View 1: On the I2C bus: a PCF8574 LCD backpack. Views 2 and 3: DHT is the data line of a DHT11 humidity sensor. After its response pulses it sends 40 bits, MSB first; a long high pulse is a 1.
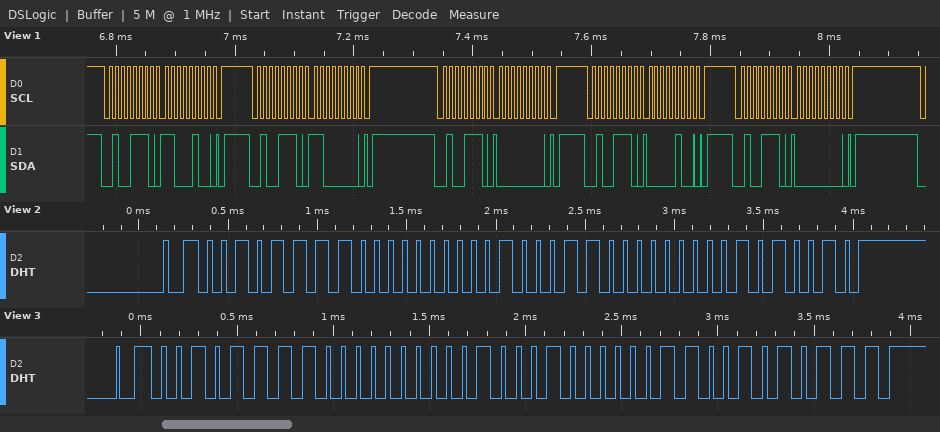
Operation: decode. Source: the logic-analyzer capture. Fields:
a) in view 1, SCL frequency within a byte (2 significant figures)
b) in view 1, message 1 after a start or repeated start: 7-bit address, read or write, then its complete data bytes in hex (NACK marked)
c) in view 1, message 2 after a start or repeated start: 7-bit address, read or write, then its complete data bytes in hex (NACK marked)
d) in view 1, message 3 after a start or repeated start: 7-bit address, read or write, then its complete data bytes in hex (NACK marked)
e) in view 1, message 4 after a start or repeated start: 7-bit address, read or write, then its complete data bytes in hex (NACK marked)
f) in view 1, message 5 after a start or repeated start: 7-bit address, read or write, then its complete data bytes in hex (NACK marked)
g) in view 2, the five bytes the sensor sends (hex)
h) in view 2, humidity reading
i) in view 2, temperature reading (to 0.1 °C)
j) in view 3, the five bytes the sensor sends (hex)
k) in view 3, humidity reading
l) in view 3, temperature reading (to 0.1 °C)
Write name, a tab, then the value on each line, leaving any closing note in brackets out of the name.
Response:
in view 1, SCL frequency within a byte	100 kHz
in view 1, message 1 after a start or repeated start: 7-bit address, read or write, then its complete data bytes in hex	0x27 write: C4
in view 1, message 2 after a start or repeated start: 7-bit address, read or write, then its complete data bytes in hex	0x27 write: C0
in view 1, message 3 after a start or repeated start: 7-bit address, read or write, then its complete data bytes in hex	0x27 write: 00
in view 1, message 4 after a start or repeated start: 7-bit address, read or write, then its complete data bytes in hex	0x27 write: 04
in view 1, message 5 after a start or repeated start: 7-bit address, read or write, then its complete data bytes in hex	0x27 write: 00
in view 2, the five bytes the sensor sends	2F 00 23 00 52
in view 2, humidity reading	47 %
in view 2, temperature reading	35.0 °C
in view 3, the five bytes the sensor sends	2F 00 22 06 57
in view 3, humidity reading	47 %
in view 3, temperature reading	34.6 °C
